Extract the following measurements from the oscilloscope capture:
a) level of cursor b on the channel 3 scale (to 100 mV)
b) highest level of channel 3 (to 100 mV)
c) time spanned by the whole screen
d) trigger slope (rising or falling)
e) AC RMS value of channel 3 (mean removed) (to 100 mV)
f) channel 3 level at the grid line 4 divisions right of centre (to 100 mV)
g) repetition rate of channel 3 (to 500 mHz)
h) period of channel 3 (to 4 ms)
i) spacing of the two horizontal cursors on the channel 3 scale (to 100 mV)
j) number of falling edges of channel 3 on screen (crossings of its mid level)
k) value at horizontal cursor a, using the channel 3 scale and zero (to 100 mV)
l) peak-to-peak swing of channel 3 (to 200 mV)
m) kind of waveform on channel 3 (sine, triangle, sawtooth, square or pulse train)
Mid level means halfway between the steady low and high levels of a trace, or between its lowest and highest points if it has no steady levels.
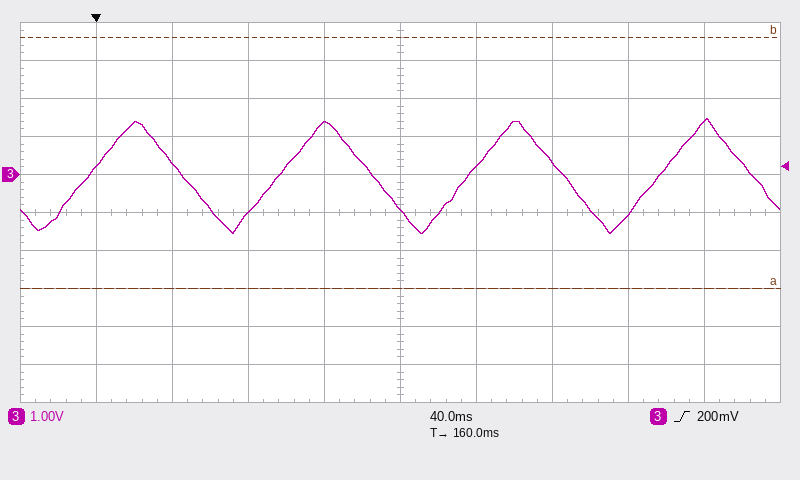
3.6 V
1.5 V
400 ms
rising
900 mV
1.4 V
10.0 Hz
100 ms
6.6 V
4
-3.0 V
3.0 V
triangle
